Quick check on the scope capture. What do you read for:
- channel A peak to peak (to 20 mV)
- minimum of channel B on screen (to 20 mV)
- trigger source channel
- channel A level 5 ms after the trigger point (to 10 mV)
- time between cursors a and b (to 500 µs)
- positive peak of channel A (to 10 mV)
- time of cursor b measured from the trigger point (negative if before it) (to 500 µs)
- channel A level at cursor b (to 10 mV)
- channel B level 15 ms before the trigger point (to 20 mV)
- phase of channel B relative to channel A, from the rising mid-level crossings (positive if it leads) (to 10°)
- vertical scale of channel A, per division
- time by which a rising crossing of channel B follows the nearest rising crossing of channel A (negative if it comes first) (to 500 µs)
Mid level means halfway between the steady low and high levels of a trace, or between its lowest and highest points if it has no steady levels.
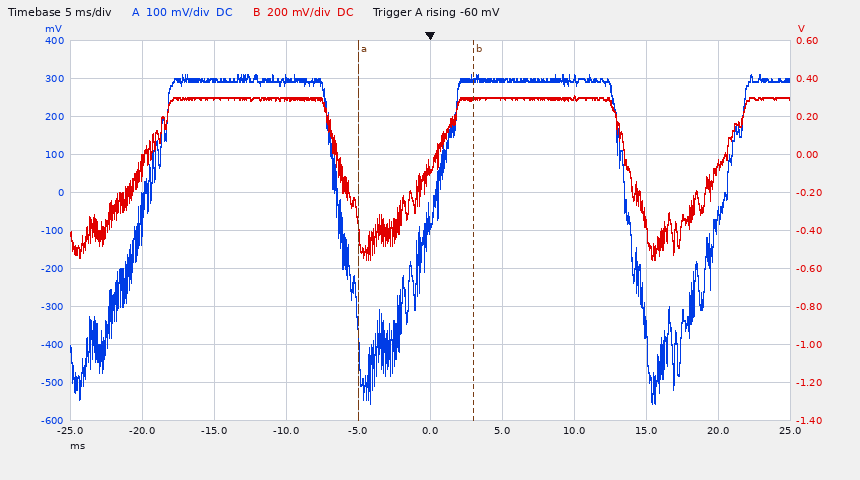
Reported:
860 mV
-560 mV
channel A
300 mV
8.0 ms
310 mV
+3.0 ms
300 mV
300 mV
0°
100 mV
0.0 ms
